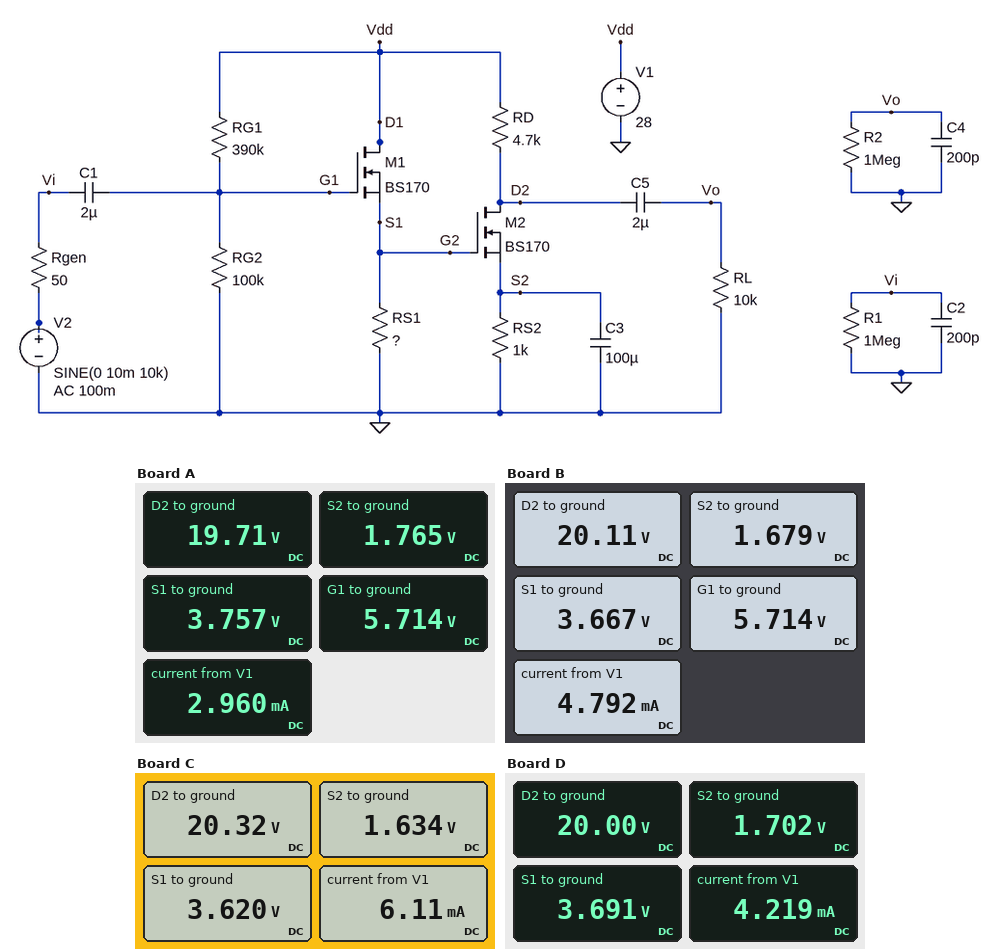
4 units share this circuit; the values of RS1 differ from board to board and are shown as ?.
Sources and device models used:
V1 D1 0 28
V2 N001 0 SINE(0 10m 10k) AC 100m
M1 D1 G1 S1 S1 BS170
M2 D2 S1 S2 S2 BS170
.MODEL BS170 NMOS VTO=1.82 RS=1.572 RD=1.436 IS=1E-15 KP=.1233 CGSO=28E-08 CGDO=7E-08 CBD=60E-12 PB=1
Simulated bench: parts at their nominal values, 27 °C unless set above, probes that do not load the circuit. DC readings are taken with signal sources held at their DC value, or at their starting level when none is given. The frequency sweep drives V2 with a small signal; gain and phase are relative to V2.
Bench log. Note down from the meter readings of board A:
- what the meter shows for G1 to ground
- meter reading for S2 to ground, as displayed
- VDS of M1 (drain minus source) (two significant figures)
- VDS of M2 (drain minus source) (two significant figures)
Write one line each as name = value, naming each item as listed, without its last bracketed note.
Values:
what the meter shows for G1 to ground = 5.714 V
meter reading for S2 to ground, as displayed = 1.765 V
VDS of M1 (drain minus source) = 24 V
VDS of M2 (drain minus source) = 18 V
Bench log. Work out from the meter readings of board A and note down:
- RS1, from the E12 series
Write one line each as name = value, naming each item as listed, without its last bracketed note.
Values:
RS1, from the E12 series = 3.3 kΩ
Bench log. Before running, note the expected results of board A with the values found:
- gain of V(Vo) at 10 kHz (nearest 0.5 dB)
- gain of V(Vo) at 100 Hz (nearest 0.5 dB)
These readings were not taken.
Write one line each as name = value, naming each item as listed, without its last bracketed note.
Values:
gain of V(Vo) at 10 kHz = 36.0 dB
gain of V(Vo) at 100 Hz = 35.5 dB
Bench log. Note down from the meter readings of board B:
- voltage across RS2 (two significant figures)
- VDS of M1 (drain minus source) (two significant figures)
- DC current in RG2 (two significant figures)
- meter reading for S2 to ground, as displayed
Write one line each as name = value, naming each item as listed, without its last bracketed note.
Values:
voltage across RS2 = 1.7 V
VDS of M1 (drain minus source) = 24 V
DC current in RG2 = 57 µA
meter reading for S2 to ground, as displayed = 1.679 V
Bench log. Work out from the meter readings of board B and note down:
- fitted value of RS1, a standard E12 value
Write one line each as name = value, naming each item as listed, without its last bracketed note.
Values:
fitted value of RS1, a standard E12 value = 1.2 kΩ
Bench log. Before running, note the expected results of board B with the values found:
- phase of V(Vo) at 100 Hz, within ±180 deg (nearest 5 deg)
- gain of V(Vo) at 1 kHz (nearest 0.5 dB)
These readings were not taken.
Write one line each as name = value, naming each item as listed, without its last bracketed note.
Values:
phase of V(Vo) at 100 Hz, within ±180 deg = -160 deg
gain of V(Vo) at 1 kHz = 35.5 dB
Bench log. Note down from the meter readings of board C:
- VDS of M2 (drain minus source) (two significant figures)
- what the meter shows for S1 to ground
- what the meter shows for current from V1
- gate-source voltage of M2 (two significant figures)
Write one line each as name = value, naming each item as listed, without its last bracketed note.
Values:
VDS of M2 (drain minus source) = 19 V
what the meter shows for S1 to ground = 3.620 V
what the meter shows for current from V1 = 6.11 mA
gate-source voltage of M2 = 2.0 V
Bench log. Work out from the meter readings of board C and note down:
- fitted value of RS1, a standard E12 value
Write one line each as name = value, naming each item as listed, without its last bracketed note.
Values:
fitted value of RS1, a standard E12 value = 820 Ω
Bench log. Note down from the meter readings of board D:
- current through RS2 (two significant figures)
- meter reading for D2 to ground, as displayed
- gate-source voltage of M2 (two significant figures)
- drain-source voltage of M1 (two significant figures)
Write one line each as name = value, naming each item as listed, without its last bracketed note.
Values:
current through RS2 = 1.7 mA
meter reading for D2 to ground, as displayed = 20.00 V
gate-source voltage of M2 = 2.0 V
drain-source voltage of M1 = 24 V
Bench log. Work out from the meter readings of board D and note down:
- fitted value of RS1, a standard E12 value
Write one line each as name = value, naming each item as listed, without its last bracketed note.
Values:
fitted value of RS1, a standard E12 value = 1.5 kΩ
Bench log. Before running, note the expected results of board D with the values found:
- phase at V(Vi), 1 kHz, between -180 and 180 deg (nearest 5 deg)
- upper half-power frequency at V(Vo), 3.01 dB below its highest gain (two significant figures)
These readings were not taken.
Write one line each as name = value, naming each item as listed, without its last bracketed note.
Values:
phase at V(Vi), 1 kHz, between -180 and 180 deg = 0 deg
upper half-power frequency at V(Vo), 3.01 dB below its highest gain = 220 kHz
